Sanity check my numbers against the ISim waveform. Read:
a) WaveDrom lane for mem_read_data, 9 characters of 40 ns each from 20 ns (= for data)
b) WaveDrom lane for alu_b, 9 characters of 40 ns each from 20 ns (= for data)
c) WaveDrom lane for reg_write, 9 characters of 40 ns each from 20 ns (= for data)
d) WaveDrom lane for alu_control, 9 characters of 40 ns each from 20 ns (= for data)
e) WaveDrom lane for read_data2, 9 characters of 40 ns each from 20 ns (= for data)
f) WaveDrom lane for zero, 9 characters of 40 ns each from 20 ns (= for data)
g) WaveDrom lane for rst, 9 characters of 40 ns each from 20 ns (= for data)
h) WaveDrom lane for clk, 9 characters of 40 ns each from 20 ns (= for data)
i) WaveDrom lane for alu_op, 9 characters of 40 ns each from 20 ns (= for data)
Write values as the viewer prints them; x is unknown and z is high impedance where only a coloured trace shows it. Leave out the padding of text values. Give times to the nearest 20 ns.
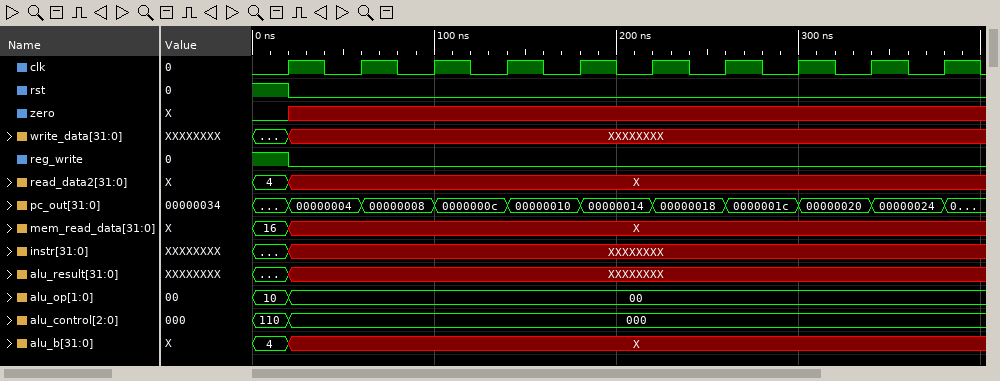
{name: 'mem_read_data', wave: 'x........'}
{name: 'alu_b', wave: 'x........'}
{name: 'reg_write', wave: '0........'}
{name: 'alu_control', wave: '=........', data: '000'}
{name: 'read_data2', wave: 'x........'}
{name: 'zero', wave: 'x........'}
{name: 'rst', wave: '0........'}
{name: 'clk', wave: 'p........'}
{name: 'alu_op', wave: '=........', data: '00'}
